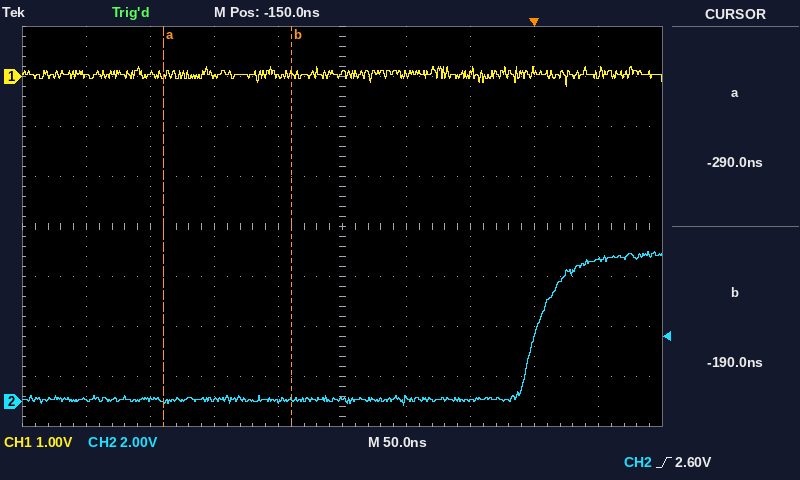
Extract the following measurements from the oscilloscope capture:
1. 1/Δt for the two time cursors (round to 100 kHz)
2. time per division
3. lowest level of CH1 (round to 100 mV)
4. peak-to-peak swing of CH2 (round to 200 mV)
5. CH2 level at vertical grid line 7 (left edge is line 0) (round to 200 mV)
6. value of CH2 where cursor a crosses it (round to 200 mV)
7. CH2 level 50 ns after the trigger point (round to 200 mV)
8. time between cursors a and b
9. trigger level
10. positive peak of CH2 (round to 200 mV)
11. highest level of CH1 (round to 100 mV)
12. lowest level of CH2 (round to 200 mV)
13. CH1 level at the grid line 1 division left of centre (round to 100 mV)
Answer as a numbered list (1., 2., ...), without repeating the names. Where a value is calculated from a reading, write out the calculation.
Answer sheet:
1. 1 / 100 ns ≈ 10.0 MHz
2. 50 ns
3. -200 mV
4. 6.0 V − (-200 mV) = 6.2 V
5. 0.0 V
6. 0.0 V
7. 5.6 V
8. -190 ns − (-290 ns) = 100 ns
9. 2.60 V
10. 6.0 V
11. 200 mV
12. -200 mV
13. 0.0 V
